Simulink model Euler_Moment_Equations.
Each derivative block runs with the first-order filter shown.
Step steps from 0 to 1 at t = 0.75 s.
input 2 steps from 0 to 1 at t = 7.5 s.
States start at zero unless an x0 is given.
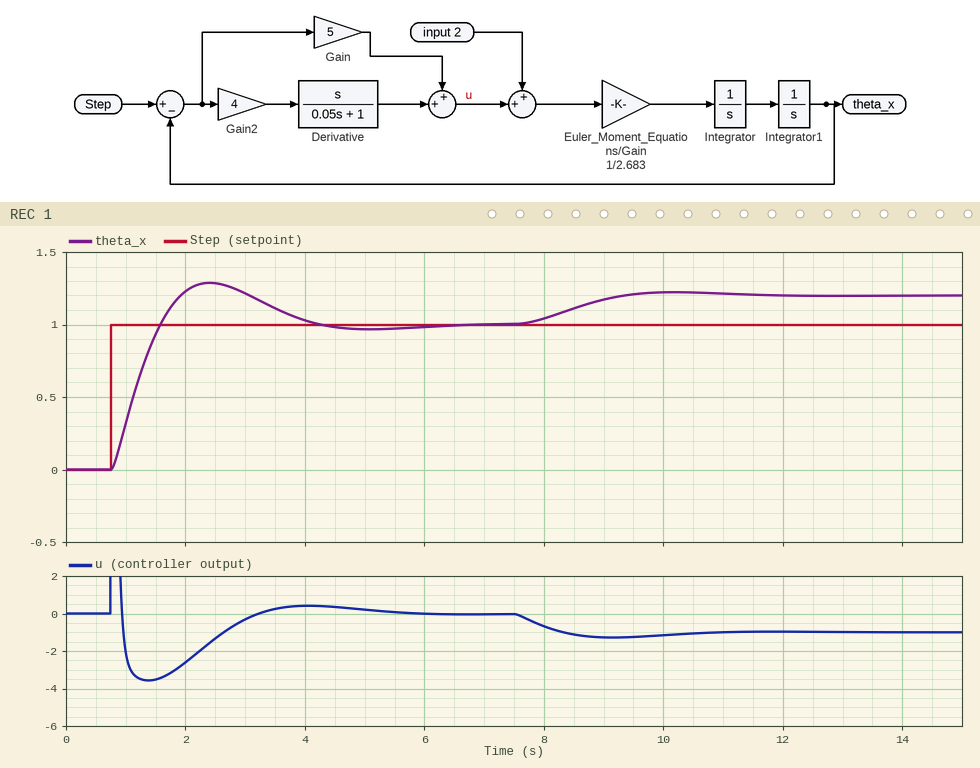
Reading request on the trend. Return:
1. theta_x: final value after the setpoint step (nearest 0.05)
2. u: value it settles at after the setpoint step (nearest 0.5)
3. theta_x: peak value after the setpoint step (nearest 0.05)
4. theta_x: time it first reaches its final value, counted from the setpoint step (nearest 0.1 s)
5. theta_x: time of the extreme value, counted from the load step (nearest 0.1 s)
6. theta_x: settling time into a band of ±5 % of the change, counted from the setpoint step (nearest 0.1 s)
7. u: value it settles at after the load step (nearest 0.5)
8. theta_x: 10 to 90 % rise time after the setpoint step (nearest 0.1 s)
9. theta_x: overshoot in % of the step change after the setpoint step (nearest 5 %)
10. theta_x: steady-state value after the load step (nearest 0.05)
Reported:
1.00
0.0
1.30
0.8 s
2.7 s
3.1 s
-1.0
0.6 s
30 %
1.20
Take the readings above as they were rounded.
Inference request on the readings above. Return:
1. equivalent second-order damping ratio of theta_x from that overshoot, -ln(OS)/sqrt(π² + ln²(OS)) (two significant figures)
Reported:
0.36
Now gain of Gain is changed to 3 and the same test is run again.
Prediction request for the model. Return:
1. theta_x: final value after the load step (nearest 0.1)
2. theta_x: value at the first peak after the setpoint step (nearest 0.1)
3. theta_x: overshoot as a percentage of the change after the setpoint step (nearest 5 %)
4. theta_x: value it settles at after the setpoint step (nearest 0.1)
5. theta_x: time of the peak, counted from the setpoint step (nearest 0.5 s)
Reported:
1.3
1.2
20 %
1.0
2.0 s
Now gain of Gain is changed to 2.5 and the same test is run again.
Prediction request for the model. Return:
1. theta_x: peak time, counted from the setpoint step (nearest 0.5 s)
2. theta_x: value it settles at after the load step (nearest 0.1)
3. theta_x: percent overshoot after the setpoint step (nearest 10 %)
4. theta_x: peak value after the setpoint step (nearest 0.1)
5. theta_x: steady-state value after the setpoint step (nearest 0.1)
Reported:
2.0 s
1.4
20 %
1.2
1.0
